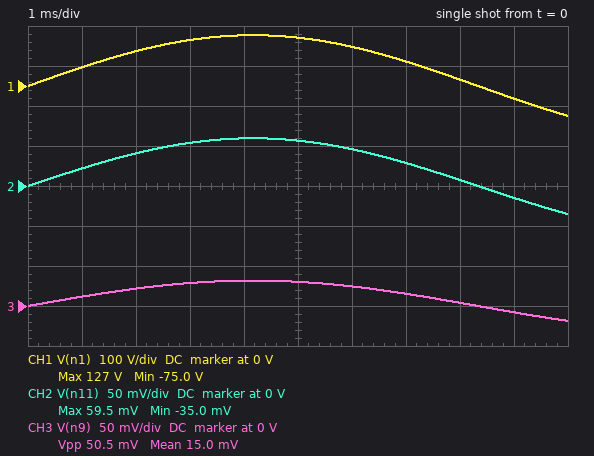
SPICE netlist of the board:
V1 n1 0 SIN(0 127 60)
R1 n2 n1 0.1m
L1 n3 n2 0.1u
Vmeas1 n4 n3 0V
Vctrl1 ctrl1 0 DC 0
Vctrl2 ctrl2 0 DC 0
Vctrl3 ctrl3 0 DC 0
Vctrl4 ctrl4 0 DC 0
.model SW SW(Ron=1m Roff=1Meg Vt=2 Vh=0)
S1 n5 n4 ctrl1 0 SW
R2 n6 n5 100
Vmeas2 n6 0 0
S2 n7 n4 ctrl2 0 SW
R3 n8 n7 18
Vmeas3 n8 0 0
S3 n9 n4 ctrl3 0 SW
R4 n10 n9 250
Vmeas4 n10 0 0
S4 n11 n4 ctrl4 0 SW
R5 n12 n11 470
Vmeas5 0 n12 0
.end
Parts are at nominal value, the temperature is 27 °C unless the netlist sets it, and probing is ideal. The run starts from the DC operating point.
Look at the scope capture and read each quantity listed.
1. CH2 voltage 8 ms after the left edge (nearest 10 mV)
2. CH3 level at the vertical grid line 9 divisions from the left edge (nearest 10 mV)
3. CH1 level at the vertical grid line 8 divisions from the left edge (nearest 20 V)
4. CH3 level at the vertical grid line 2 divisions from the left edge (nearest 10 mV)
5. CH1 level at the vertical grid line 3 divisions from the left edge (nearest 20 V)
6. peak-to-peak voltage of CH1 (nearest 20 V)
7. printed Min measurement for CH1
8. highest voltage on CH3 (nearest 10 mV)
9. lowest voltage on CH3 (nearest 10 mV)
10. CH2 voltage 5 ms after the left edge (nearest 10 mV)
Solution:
10 mV
-10 mV
20 V
20 mV
120 V
200 V
-75.0 V
30 mV
-20 mV
60 mV
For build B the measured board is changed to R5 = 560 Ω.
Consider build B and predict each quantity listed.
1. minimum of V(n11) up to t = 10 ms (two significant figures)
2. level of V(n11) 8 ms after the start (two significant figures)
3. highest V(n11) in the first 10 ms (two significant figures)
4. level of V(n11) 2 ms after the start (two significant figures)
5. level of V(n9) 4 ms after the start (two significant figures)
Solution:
-42 mV
8.9 mV
71 mV
49 mV
32 mV
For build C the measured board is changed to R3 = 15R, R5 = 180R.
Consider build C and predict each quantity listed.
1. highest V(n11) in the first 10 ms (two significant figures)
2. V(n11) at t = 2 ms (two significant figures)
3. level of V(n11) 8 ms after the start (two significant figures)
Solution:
23 mV
16 mV
2.9 mV
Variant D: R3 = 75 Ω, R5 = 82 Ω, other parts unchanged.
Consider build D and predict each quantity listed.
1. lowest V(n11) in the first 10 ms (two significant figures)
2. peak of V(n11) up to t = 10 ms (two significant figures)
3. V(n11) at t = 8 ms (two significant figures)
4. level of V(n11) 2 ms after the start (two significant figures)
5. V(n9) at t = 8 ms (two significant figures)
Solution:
-6.1 mV
10 mV
1.3 mV
7.1 mV
4.0 mV
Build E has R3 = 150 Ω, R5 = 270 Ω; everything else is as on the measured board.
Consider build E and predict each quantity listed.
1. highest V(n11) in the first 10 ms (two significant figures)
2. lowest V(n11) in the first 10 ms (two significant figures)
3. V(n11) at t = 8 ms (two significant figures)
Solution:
34 mV
-20 mV
4.3 mV
